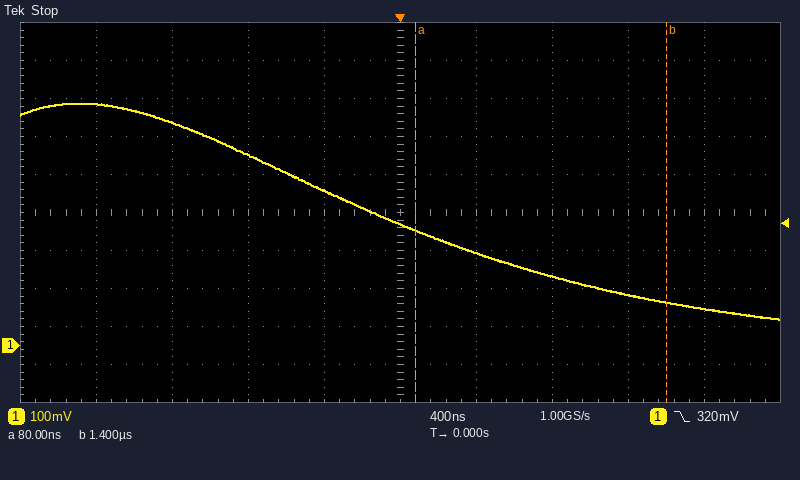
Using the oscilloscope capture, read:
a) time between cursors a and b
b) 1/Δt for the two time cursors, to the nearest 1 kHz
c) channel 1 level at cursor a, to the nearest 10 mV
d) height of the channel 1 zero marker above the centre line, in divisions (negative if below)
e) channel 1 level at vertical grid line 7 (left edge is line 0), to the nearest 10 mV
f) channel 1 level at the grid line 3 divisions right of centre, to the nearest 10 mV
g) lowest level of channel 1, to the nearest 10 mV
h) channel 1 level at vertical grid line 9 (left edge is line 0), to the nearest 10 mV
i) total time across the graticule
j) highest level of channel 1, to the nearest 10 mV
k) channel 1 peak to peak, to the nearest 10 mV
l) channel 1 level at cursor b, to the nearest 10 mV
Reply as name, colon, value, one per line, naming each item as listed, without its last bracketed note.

time between cursors a and b: 1.32 µs
1/Δt for the two time cursors, to the nearest 1 kHz: 758 kHz
channel 1 level at cursor a, to the nearest 10 mV: 300 mV
height of the channel 1 zero marker above the centre line, in divisions: -3.5 div
channel 1 level at vertical grid line 7 (left edge is line 0), to the nearest 10 mV: 180 mV
channel 1 level at the grid line 3 divisions right of centre, to the nearest 10 mV: 130 mV
lowest level of channel 1, to the nearest 10 mV: 70 mV
channel 1 level at vertical grid line 9 (left edge is line 0), to the nearest 10 mV: 100 mV
total time across the graticule: 4 µs
highest level of channel 1, to the nearest 10 mV: 640 mV
channel 1 peak to peak, to the nearest 10 mV: 570 mV
channel 1 level at cursor b, to the nearest 10 mV: 110 mV
